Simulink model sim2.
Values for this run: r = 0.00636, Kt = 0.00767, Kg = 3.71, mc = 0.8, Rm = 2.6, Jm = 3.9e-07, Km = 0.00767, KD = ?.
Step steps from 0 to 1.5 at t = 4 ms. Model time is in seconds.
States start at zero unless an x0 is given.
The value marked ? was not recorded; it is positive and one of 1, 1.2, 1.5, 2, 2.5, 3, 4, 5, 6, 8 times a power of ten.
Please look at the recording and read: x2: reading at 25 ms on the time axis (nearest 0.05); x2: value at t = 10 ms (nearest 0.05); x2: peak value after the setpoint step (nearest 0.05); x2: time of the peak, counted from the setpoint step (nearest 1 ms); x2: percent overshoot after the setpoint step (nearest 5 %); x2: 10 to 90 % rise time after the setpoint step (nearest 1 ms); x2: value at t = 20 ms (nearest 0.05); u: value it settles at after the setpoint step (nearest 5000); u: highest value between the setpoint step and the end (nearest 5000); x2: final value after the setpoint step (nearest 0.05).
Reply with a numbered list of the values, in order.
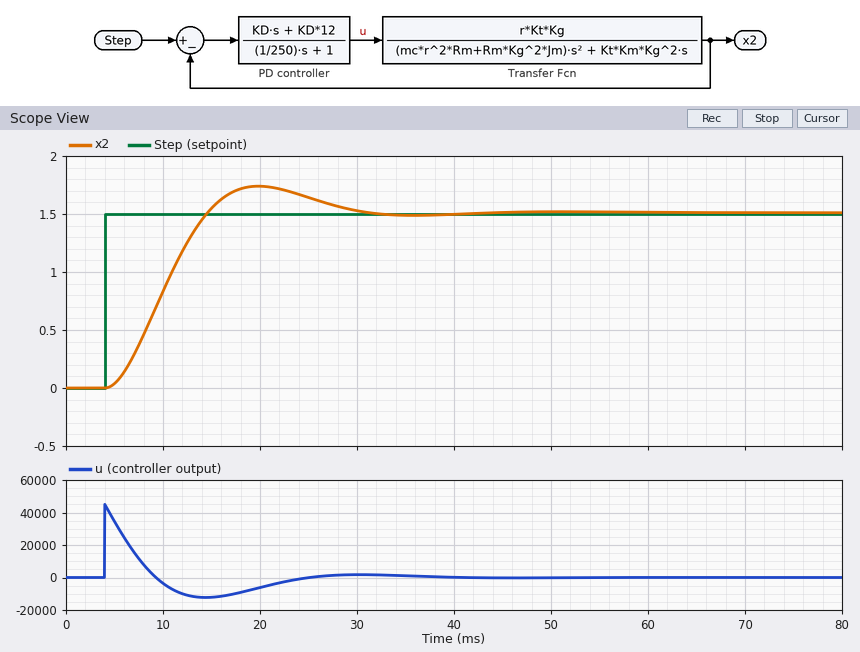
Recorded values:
1. 1.65
2. 0.85
3. 1.75
4. 16 ms
5. 15 %
6. 7 ms
7. 1.75
8. 0
9. 45000
10. 1.50
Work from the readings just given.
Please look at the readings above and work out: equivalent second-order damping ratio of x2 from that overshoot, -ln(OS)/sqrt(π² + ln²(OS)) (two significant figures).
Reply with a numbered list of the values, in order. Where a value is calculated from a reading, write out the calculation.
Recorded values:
1. ln(0.15) = -1.897; 1.897 / sqrt(9.870 + 3.599) = 0.52
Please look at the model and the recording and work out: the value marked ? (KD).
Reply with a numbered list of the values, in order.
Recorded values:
1. 120
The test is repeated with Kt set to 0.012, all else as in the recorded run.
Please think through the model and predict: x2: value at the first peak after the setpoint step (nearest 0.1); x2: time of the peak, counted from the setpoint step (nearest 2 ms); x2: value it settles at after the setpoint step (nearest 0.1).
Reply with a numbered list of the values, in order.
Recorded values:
1. 1.8
2. 12 ms
3. 1.5
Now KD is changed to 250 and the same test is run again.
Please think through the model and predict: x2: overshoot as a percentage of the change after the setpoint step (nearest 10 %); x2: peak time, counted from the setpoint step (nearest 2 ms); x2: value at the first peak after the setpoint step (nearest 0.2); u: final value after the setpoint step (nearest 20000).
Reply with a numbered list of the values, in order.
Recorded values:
1. 30 %
2. 10 ms
3. 2.0
4. 0
